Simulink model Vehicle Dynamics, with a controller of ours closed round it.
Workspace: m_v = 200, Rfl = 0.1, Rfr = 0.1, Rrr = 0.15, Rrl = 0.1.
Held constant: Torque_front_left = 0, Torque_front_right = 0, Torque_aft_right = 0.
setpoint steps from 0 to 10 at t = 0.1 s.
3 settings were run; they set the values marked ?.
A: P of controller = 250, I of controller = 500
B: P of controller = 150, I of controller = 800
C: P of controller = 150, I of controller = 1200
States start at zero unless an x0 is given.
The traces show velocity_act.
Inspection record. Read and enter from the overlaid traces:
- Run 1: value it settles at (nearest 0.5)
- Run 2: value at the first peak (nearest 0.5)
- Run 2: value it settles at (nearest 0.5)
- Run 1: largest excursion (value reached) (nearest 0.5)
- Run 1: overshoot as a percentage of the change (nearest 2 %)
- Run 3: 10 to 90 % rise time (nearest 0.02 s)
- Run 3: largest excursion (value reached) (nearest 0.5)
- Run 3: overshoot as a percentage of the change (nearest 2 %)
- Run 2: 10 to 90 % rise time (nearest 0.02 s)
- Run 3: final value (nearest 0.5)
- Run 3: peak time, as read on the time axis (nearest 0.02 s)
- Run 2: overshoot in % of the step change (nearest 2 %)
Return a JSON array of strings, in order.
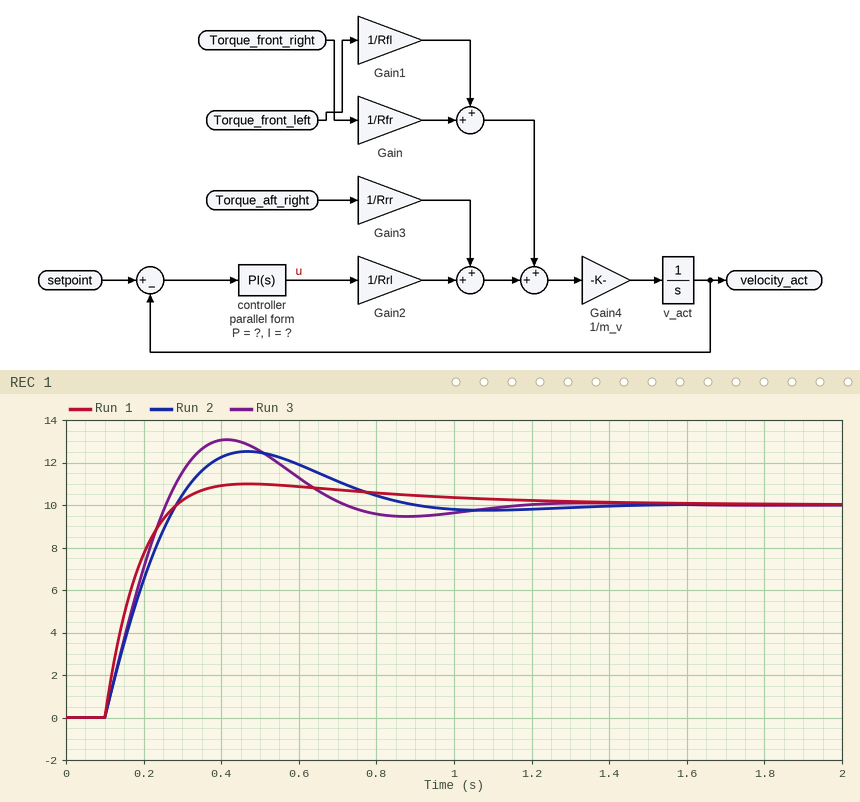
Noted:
["10.0", "12.5", "10.0", "11.0", "10 %", "0.12 s", "13.0", "30 %", "0.14 s", "10.0", "0.42 s", "26 %"]
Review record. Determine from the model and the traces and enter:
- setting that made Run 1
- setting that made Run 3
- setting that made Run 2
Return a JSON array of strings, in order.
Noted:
["A", "C", "B"]
